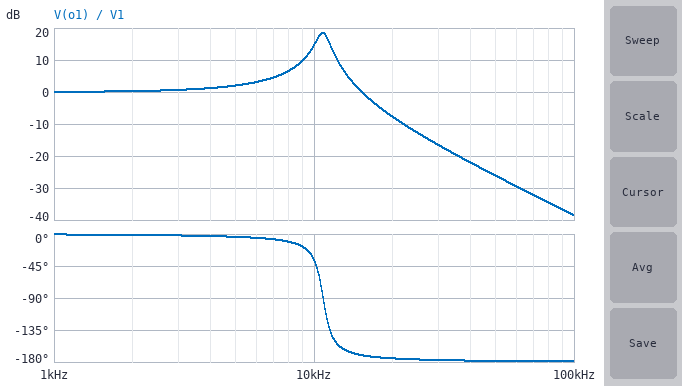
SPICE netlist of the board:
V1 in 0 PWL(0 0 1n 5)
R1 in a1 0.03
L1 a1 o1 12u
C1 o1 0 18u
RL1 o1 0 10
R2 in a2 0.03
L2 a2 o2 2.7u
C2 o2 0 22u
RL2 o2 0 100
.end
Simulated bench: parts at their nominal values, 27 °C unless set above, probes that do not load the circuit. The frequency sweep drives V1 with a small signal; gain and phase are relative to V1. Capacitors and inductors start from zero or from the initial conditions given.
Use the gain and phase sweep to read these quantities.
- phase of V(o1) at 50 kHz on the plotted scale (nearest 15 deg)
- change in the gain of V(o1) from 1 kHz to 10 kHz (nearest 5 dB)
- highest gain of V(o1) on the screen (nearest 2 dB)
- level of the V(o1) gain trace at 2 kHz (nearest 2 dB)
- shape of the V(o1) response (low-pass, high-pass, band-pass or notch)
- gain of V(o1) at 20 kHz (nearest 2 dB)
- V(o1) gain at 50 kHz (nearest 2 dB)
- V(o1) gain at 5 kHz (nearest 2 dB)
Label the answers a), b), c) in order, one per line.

a) -180 deg
b) 15 dB
c) 18 dB
d) 0 dB
e) low-pass
f) -8 dB
g) -26 dB
h) 2 dB
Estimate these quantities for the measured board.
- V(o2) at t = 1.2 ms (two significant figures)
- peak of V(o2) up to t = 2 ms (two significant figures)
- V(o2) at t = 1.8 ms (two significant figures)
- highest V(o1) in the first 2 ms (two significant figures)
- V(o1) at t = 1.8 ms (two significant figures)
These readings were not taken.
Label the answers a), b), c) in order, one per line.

a) 5.0 V
b) 9.3 V
c) 5.0 V
d) 9.1 V
e) 5.0 V
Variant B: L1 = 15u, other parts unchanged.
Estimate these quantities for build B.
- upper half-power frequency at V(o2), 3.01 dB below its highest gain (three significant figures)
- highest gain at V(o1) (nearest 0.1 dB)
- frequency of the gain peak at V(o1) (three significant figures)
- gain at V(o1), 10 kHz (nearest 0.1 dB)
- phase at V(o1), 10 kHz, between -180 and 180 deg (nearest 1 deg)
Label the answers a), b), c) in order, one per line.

a) 21.5 kHz
b) 18.1 dB
c) 9.66 kHz
d) 16.9 dB
e) -116 deg
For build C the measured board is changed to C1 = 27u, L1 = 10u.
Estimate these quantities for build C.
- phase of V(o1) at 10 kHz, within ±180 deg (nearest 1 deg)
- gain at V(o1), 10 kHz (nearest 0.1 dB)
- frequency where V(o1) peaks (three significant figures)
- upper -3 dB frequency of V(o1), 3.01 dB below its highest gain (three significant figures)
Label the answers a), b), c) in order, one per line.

a) -119 deg
b) 17.7 dB
c) 9.67 kHz
d) 10.2 kHz
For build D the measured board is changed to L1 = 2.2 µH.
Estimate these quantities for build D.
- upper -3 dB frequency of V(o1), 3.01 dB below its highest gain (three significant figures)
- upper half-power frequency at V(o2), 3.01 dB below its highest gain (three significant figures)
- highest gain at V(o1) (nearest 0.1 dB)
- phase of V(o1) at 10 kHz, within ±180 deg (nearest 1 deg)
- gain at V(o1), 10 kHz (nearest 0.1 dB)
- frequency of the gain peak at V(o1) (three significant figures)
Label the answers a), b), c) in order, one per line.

a) 26.7 kHz
b) 21.5 kHz
c) 18.4 dB
d) -3 deg
e) 1.4 dB
f) 25.2 kHz
